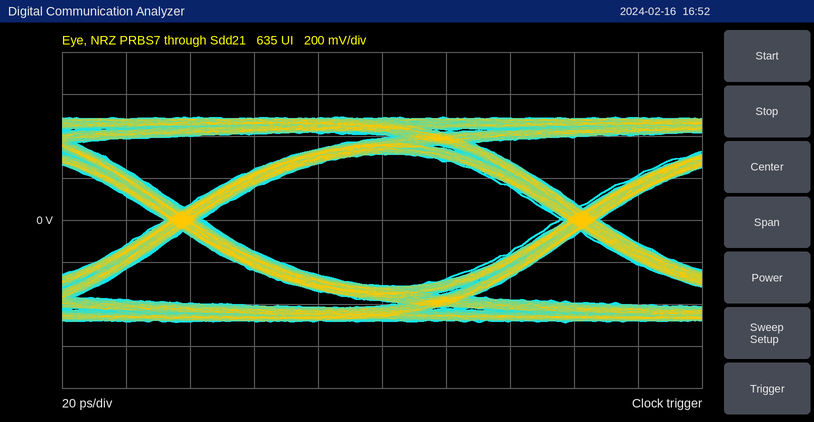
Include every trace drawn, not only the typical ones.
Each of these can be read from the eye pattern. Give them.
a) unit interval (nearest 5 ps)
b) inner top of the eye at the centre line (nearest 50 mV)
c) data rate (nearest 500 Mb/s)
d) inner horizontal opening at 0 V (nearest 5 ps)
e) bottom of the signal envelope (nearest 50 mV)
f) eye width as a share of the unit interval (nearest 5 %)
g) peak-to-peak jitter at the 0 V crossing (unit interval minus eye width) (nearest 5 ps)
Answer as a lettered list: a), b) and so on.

a) 125 ps
b) 300 mV
c) 8.0 Gb/s
d) 110 ps
e) -500 mV
f) 90 %
g) 15 ps
